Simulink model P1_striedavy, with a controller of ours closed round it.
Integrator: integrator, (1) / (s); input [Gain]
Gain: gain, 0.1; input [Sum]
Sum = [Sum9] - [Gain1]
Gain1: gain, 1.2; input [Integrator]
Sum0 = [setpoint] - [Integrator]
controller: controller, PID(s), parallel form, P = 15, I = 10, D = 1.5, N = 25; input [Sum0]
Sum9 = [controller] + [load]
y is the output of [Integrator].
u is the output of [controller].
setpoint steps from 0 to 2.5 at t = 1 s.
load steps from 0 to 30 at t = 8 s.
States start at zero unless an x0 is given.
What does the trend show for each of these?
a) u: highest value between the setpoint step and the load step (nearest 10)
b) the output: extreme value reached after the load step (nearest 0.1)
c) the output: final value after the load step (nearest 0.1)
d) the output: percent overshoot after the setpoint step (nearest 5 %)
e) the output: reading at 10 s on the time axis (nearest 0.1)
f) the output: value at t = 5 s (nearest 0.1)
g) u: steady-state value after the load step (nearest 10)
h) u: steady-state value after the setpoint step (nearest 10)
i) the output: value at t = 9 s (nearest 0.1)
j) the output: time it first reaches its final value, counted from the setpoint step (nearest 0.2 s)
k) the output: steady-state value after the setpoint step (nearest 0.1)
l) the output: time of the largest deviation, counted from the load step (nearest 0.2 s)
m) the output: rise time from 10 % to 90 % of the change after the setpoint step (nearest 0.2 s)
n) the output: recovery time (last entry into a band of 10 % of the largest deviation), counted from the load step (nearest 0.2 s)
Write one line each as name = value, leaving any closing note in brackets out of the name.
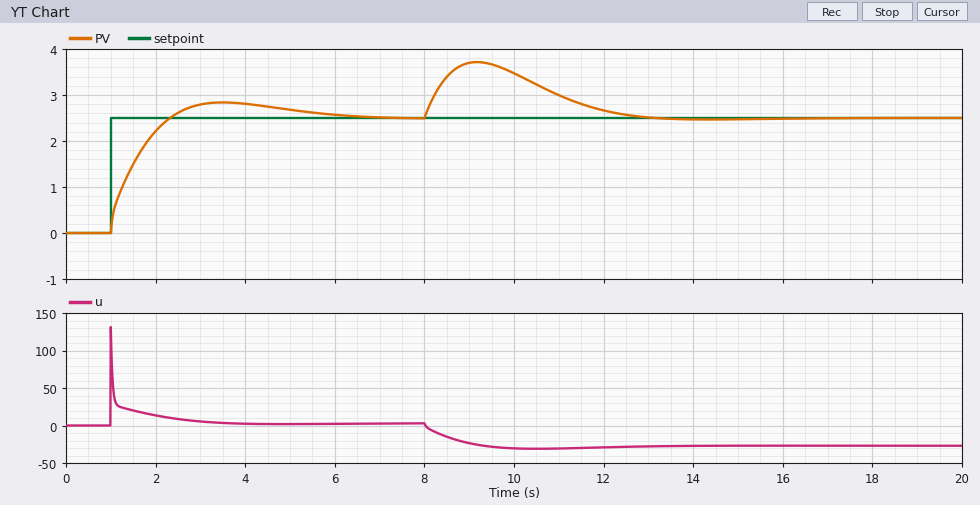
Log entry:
u: highest value between the setpoint step and the load step = 130
the output: extreme value reached after the load step = 3.7
the output: final value after the load step = 2.5
the output: percent overshoot after the setpoint step = 15 %
the output: reading at 10 s on the time axis = 3.5
the output: value at t = 5 s = 2.7
u: steady-state value after the load step = -30
u: steady-state value after the setpoint step = 0
the output: value at t = 9 s = 3.7
the output: time it first reaches its final value, counted from the setpoint step = 1.4 s
the output: steady-state value after the setpoint step = 2.5
the output: time of the largest deviation, counted from the load step = 1.2 s
the output: rise time from 10 % to 90 % of the change after the setpoint step = 1.0 s
the output: recovery time (last entry into a band of 10 % of the largest deviation), counted from the load step = 4.2 s
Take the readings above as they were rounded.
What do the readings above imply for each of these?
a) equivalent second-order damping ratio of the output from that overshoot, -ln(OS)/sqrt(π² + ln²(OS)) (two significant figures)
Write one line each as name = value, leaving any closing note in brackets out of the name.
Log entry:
equivalent second-order damping ratio of the output from that overshoot, -ln(OS)/sqrt(π² + ln²(OS)) = 0.52
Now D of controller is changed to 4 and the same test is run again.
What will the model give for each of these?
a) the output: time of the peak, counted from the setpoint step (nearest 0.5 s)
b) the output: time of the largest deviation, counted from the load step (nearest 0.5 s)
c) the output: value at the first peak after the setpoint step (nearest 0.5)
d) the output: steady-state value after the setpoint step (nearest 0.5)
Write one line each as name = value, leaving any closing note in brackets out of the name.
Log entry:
the output: time of the peak, counted from the setpoint step = 3.0 s
the output: time of the largest deviation, counted from the load step = 1.5 s
the output: value at the first peak after the setpoint step = 3.0
the output: steady-state value after the setpoint step = 2.5
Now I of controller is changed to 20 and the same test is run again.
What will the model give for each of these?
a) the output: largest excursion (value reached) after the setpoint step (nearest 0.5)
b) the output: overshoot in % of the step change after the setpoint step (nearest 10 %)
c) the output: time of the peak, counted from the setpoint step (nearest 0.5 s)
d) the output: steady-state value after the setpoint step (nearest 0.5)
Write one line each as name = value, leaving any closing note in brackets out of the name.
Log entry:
the output: largest excursion (value reached) after the setpoint step = 3.0
the output: overshoot in % of the step change after the setpoint step = 20 %
the output: time of the peak, counted from the setpoint step = 2.0 s
the output: steady-state value after the setpoint step = 2.5
